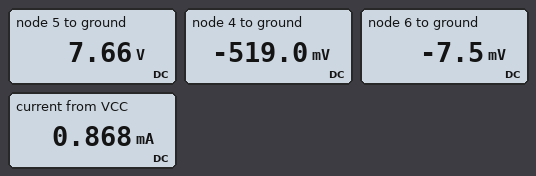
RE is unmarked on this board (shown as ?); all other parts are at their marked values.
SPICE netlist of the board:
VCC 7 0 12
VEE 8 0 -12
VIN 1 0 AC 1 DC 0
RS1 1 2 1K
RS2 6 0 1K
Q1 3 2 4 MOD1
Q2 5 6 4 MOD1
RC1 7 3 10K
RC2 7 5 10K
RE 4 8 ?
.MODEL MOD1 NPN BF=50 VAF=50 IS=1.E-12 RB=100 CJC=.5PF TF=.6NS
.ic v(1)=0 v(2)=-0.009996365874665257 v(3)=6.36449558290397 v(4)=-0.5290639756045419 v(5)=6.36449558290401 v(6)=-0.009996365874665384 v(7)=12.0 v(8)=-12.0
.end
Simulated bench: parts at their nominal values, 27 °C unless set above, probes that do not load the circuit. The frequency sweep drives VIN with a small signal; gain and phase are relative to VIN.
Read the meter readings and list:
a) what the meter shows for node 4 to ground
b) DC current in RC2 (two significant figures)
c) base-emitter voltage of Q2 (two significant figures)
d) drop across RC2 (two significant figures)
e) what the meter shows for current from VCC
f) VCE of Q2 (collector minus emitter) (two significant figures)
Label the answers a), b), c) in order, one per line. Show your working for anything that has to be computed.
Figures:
a) -519.0 mV
b) (12 V - 7.66 V) / 10 kΩ = 430 µA
c) -7.5 mV - (-519 mV) = 510 mV
d) 12 V - 7.66 V = 4.3 V
e) 0.868 mA
f) 7.66 V - (-519 mV) = 8.2 V
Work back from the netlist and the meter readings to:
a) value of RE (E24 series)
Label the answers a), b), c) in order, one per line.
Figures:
a) 13 kΩ
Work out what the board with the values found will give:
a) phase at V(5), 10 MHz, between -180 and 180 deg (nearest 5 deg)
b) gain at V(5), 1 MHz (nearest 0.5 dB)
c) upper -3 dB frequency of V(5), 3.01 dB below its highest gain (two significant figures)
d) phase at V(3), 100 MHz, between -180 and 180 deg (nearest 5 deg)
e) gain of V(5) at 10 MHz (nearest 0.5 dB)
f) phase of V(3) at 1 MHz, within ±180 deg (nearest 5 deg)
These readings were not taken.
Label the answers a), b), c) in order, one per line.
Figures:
a) -70 deg
b) 35.0 dB
c) 4.1 MHz
d) 70 deg
e) 27.0 dB
f) 165 deg
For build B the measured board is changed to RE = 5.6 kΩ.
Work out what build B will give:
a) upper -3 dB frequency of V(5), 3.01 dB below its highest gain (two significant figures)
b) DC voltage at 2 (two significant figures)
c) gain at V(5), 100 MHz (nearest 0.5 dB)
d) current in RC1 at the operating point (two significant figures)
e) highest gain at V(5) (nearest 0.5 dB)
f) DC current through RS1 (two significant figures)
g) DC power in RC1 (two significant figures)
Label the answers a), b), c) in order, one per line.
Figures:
a) 2.0 MHz
b) -19 mV
c) 3.0 dB
d) 1.0 mA
e) 39.0 dB
f) 19 µA
g) 10 mW
